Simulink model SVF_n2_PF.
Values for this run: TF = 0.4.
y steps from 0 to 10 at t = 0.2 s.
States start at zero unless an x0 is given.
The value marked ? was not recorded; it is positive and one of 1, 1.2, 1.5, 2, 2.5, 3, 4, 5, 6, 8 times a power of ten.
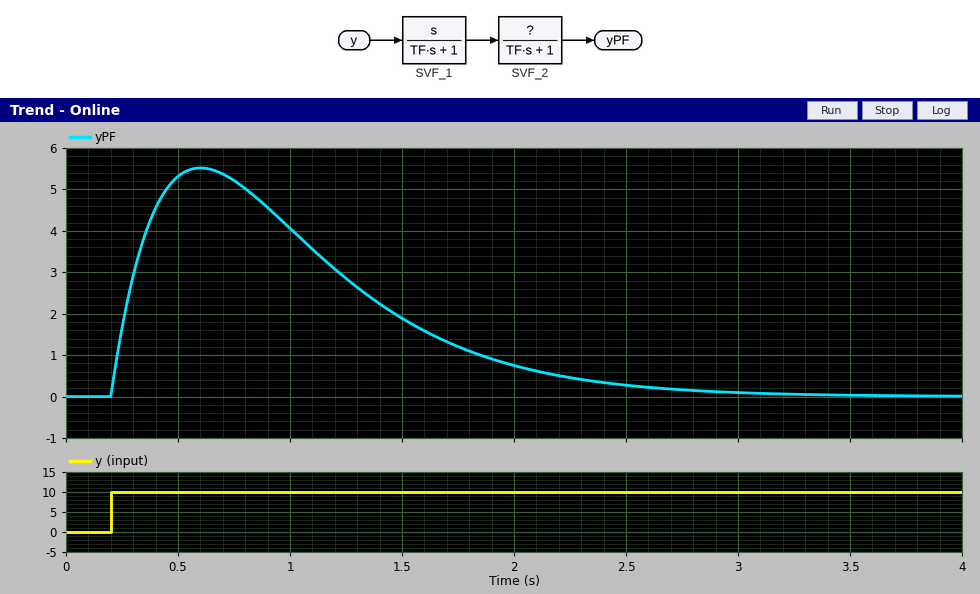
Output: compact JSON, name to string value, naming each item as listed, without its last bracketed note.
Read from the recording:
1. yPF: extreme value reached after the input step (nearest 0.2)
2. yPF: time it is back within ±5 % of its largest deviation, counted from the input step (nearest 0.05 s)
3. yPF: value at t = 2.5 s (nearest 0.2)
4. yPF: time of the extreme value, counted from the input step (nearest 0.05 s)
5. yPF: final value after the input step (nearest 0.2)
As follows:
{"yPF: extreme value reached after the input step": "5.6", "yPF: time it is back within ±5 % of its largest deviation, counted from the input step": "2.30 s", "yPF: value at t = 2.5 s": "0.2", "yPF: time of the extreme value, counted from the input step": "0.40 s", "yPF: final value after the input step": "0.0"}
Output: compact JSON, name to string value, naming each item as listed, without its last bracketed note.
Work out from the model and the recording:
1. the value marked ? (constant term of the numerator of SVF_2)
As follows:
{"the value marked ?": "0.6"}
